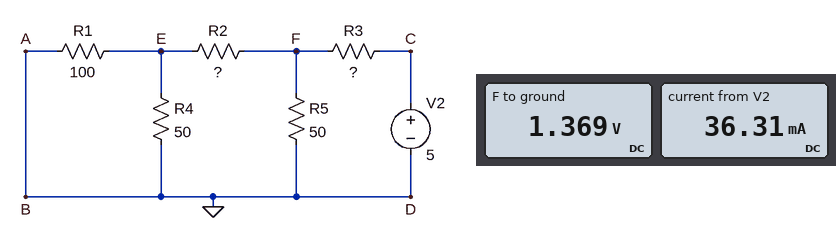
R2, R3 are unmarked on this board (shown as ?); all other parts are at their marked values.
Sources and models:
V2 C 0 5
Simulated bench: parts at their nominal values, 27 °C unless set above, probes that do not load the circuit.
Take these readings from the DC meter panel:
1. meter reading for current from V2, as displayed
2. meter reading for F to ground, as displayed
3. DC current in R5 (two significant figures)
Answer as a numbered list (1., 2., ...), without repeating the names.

1. 36.31 mA
2. 1.369 V
3. 27 mA
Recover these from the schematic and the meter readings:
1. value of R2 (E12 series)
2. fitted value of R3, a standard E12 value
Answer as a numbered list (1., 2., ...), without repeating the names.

1. 120 Ω
2. 100 Ω
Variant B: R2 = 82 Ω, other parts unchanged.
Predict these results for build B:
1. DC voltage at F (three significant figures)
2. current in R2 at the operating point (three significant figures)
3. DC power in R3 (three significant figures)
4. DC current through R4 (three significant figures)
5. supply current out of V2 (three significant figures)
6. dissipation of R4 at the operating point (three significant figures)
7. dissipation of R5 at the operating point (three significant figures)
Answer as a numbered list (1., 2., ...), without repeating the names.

1. 1.29 V
2. 11.2 mA
3. 137 mW
4. 7.47 mA
5. 37.1 mA
6. 2.79 mW
7. 33.4 mW
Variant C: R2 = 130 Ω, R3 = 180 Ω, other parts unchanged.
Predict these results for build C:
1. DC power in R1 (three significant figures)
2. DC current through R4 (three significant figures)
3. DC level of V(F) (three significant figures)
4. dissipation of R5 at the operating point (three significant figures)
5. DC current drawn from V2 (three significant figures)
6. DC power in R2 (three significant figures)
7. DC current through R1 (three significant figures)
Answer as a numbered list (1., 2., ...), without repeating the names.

1. 320 µW
2. 3.58 mA
3. 877 mV
4. 15.4 mW
5. 22.9 mA
6. 3.75 mW
7. 1.79 mA
